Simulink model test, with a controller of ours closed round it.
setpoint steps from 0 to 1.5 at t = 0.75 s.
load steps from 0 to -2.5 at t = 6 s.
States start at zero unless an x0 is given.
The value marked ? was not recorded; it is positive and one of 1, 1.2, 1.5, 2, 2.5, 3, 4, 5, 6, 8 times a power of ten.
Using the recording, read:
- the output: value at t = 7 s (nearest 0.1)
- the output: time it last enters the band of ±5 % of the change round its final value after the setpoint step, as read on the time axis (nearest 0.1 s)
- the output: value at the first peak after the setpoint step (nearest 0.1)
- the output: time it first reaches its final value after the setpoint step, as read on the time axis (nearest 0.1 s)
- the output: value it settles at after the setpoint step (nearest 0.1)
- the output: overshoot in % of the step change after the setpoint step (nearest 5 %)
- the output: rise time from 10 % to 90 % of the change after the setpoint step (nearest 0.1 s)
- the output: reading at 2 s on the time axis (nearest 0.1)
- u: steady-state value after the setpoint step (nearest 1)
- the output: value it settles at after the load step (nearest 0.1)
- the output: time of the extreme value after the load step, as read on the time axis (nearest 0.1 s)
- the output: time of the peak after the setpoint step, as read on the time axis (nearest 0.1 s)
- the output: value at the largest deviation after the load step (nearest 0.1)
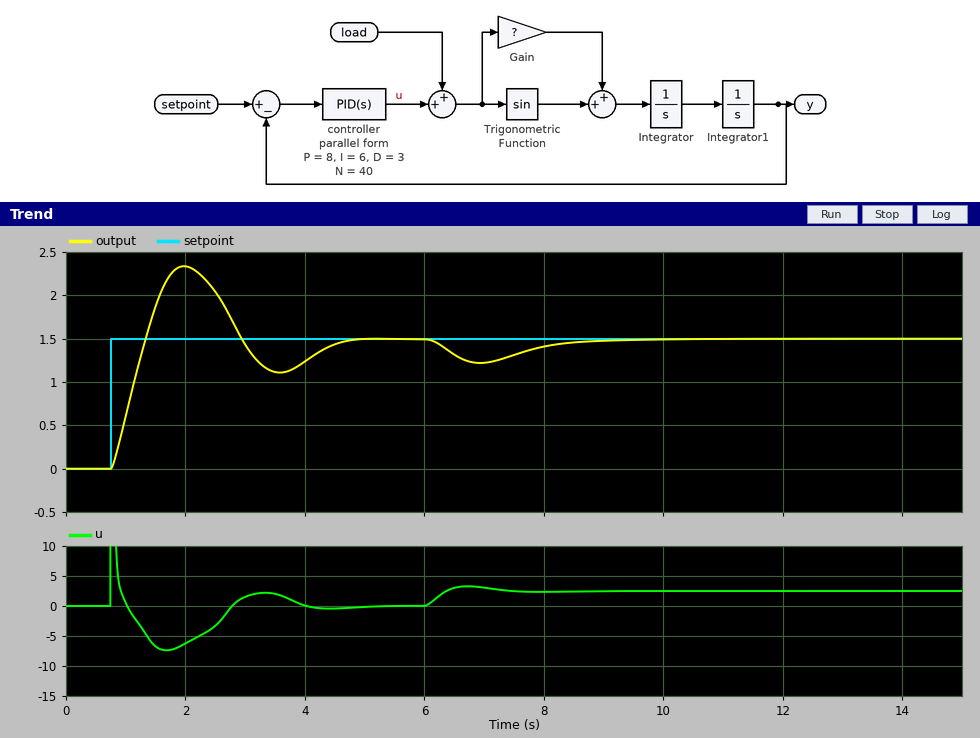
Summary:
1.2
4.5 s
2.3
1.3 s
1.5
55 %
0.4 s
2.3
0
1.5
6.9 s
2.0 s
1.2
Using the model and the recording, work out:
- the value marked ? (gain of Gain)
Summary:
0.5
